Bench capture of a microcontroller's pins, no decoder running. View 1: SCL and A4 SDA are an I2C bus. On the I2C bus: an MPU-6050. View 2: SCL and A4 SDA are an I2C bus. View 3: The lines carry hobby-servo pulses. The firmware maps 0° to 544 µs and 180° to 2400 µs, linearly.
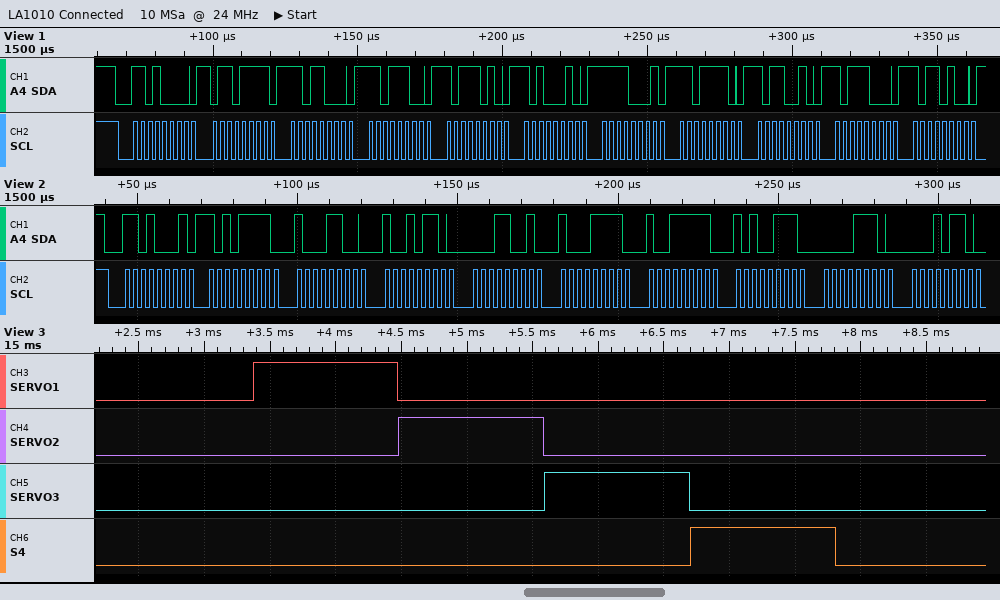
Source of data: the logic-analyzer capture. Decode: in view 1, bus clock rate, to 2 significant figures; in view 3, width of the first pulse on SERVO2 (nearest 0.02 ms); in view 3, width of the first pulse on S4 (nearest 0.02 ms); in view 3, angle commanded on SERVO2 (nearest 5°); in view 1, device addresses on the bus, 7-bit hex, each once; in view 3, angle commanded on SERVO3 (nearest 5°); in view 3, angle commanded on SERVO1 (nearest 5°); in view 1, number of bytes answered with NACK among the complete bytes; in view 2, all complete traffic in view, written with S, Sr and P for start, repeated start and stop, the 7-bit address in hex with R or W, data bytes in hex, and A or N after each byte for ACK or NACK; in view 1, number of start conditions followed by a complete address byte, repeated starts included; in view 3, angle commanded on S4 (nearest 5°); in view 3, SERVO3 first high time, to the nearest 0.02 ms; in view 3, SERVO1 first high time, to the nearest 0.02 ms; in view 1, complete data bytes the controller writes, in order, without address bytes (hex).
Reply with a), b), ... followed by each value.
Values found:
a) 400 kHz
b) 1.10 ms
c) 1.10 ms
d) 55°
e) 0x68
f) 55°
g) 55°
h) 0
i) S 68R A AF A 8C A 96 A 19 A 8F A 9F A A7 A 0E A 16 A
j) 1
k) 55°
l) 1.10 ms
m) 1.10 ms
n) 6F D8 DC BA A2 F1 DE B2 B8 B4
